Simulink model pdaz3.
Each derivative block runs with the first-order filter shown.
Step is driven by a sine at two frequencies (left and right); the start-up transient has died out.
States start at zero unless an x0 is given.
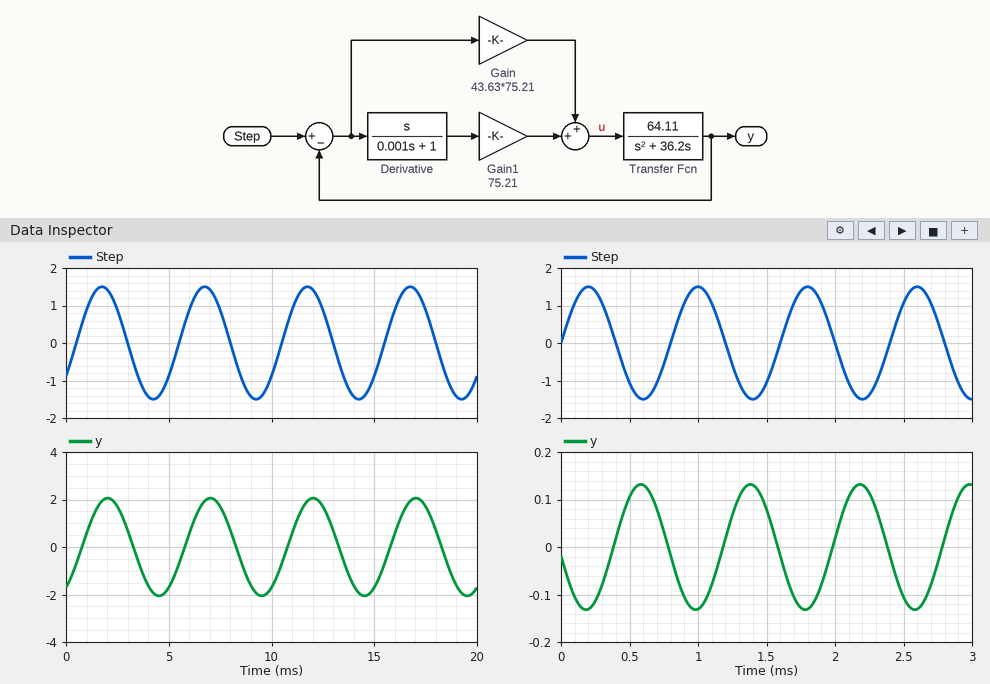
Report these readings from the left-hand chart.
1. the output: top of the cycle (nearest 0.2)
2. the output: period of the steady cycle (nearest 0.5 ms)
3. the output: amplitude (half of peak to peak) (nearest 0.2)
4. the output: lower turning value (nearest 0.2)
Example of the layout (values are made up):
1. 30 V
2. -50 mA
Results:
1. 2.0
2. 5.0 ms
3. 2.0
4. -2.0
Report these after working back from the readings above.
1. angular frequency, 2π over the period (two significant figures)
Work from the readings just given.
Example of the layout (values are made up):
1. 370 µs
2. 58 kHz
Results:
1. 1.3 rad/ms
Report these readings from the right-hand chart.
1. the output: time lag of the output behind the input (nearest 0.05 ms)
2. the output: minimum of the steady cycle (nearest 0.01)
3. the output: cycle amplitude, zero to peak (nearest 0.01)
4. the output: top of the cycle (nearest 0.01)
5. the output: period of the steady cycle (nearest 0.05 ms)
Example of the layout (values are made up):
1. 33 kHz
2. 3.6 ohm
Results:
1. 0.40 ms
2. -0.13
3. 0.13
4. 0.13
5. 0.80 ms
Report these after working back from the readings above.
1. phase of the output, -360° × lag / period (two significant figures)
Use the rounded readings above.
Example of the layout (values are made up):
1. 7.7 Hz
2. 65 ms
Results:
1. -180°
